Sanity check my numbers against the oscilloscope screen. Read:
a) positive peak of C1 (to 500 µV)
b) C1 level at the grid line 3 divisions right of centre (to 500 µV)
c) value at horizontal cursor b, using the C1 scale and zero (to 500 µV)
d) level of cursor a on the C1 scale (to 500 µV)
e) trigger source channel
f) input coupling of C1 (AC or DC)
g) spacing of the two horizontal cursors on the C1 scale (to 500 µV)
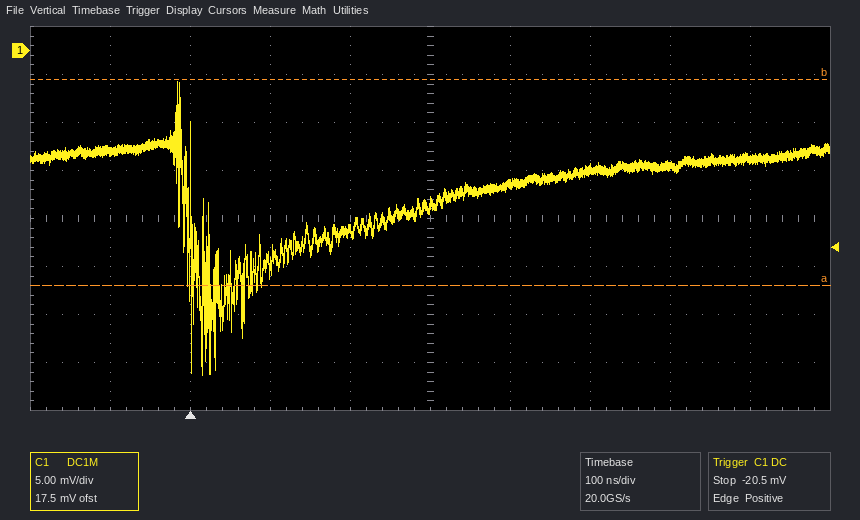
-3.0 mV
-12.0 mV
-3.0 mV
-24.5 mV
C1
DC
21.5 mV
